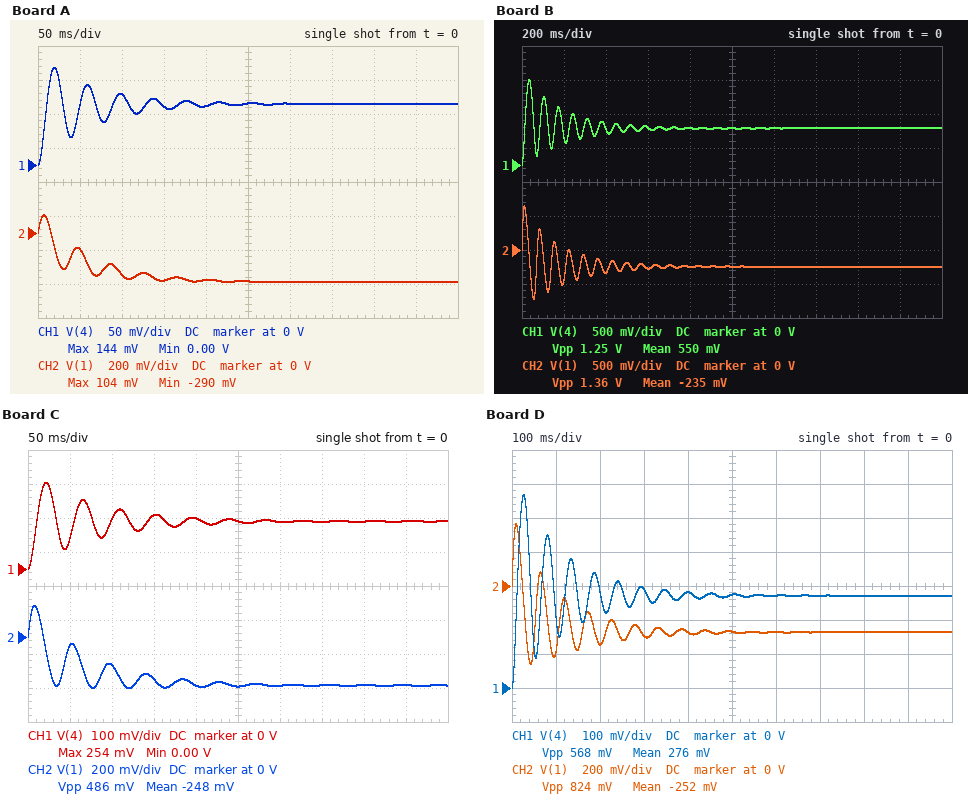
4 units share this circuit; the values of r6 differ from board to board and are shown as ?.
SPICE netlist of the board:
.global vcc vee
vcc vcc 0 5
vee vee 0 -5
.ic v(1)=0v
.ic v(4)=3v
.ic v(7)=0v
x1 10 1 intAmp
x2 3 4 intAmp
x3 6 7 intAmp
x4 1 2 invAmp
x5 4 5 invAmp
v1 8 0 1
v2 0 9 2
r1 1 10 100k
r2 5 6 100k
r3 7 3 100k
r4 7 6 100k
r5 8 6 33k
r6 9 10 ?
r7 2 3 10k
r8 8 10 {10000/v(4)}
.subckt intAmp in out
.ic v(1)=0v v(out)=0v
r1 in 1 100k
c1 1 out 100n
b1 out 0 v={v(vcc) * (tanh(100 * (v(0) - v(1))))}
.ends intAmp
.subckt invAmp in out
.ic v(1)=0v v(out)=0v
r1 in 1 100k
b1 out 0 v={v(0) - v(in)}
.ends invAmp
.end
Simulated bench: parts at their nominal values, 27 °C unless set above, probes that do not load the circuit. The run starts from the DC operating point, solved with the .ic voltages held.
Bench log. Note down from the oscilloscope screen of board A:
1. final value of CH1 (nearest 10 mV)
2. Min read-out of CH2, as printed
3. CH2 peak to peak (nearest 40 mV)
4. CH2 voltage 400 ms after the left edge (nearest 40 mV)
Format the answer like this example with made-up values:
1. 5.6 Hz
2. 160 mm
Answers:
1. 90 mV
2. -290 mV
3. 400 mV
4. -280 mV
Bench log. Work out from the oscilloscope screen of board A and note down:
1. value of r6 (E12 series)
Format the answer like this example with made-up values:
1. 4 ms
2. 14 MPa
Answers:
1. 330 kΩ
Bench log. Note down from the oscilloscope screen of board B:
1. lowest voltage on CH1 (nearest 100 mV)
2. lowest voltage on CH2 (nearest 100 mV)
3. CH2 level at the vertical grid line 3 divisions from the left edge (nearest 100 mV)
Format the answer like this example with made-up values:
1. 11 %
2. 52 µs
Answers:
1. 0 V
2. -700 mV
3. -300 mV
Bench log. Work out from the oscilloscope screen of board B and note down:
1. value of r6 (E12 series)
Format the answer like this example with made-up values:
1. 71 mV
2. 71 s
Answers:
1. 39 kΩ
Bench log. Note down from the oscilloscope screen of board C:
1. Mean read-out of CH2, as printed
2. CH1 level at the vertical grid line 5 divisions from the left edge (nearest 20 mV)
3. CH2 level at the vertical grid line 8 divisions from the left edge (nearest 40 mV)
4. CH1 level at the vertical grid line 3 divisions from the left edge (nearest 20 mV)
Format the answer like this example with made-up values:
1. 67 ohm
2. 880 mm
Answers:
1. -248 mV
2. 140 mV
3. -280 mV
4. 160 mV
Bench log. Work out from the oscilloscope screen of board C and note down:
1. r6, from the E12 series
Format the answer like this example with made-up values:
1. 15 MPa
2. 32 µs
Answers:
1. 180 kΩ
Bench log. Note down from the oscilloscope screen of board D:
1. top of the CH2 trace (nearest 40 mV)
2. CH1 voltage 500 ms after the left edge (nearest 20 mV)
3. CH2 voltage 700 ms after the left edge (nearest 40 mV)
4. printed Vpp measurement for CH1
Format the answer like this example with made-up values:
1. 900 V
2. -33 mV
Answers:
1. 360 mV
2. 280 mV
3. -280 mV
4. 568 mV
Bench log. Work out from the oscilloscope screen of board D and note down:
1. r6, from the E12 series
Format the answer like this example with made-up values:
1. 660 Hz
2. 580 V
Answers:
1. 82 kΩ
